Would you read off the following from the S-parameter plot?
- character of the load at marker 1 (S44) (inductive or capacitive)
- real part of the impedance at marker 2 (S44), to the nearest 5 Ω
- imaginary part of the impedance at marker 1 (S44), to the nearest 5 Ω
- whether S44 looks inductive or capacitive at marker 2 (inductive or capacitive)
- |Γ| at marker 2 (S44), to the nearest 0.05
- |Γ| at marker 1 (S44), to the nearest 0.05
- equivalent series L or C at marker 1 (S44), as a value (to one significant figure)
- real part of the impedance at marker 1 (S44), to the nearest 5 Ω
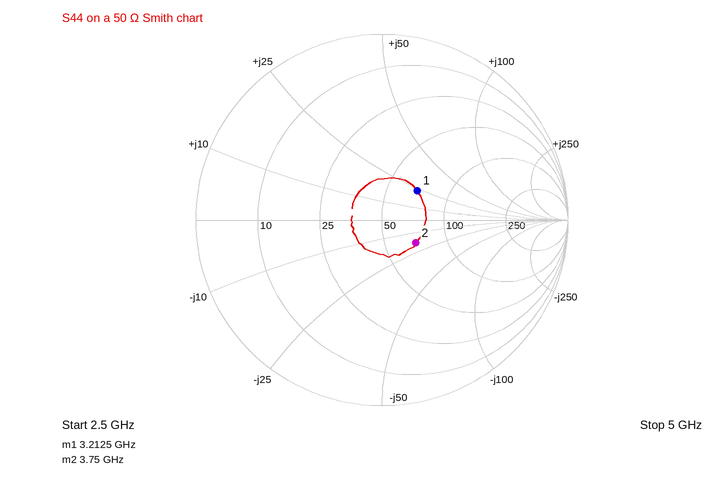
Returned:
inductive
70 Ω
+25 Ω
capacitive
0.20
0.25
1 nH
70 Ω
